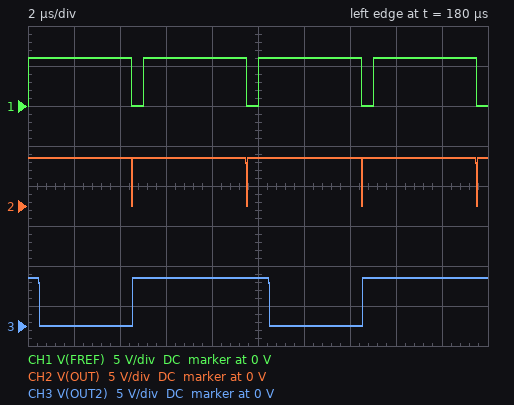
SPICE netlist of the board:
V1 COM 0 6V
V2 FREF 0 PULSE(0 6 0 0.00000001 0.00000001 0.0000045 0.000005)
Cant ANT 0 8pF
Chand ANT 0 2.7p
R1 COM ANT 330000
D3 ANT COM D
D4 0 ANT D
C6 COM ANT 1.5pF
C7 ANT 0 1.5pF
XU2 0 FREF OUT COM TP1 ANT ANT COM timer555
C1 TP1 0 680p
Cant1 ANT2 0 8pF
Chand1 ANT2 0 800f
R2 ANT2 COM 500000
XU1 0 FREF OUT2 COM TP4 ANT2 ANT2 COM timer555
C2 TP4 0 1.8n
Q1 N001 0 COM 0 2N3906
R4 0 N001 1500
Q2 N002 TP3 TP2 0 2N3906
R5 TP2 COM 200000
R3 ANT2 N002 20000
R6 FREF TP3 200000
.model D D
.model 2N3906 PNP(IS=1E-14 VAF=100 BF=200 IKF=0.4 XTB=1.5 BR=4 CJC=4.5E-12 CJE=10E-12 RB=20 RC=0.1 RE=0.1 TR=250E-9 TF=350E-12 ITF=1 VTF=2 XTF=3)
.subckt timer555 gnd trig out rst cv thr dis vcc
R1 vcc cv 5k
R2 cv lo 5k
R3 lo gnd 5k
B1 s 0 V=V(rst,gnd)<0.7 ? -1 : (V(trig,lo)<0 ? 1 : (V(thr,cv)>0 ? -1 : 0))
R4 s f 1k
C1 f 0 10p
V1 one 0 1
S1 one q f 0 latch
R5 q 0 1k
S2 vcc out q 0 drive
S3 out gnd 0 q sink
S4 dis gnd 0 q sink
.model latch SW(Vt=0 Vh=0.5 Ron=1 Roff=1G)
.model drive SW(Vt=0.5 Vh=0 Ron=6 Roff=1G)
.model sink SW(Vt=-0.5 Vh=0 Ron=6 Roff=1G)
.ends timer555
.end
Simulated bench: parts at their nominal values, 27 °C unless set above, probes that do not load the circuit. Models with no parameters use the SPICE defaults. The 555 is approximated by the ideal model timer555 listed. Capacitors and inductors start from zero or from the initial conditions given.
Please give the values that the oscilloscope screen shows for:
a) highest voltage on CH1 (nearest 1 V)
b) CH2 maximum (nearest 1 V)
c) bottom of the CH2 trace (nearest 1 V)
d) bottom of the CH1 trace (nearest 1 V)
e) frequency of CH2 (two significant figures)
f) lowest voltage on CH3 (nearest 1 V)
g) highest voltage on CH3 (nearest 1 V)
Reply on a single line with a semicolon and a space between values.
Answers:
6 V; 6 V; 0 V; 0 V; 200 kHz; 0 V; 6 V
